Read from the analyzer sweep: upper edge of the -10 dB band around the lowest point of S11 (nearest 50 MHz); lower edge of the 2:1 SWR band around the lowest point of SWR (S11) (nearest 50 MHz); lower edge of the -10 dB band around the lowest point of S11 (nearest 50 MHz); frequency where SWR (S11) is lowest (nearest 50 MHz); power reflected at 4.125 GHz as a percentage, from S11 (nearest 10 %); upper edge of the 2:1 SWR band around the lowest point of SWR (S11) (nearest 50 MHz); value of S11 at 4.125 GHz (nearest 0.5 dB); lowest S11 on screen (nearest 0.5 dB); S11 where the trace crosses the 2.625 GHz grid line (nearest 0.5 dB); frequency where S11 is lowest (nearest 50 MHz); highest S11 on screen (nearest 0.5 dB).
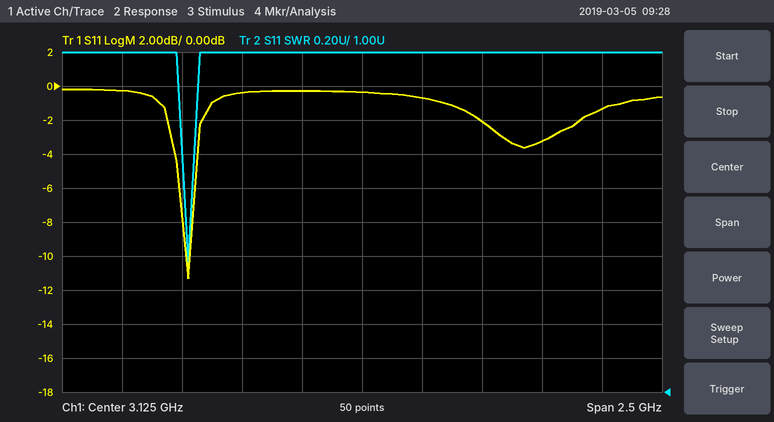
2.40 GHz
2.40 GHz
2.40 GHz
2.40 GHz
70 %
2.40 GHz
-1.5 dB
-11.5 dB
-0.5 dB
2.40 GHz
0.0 dB
